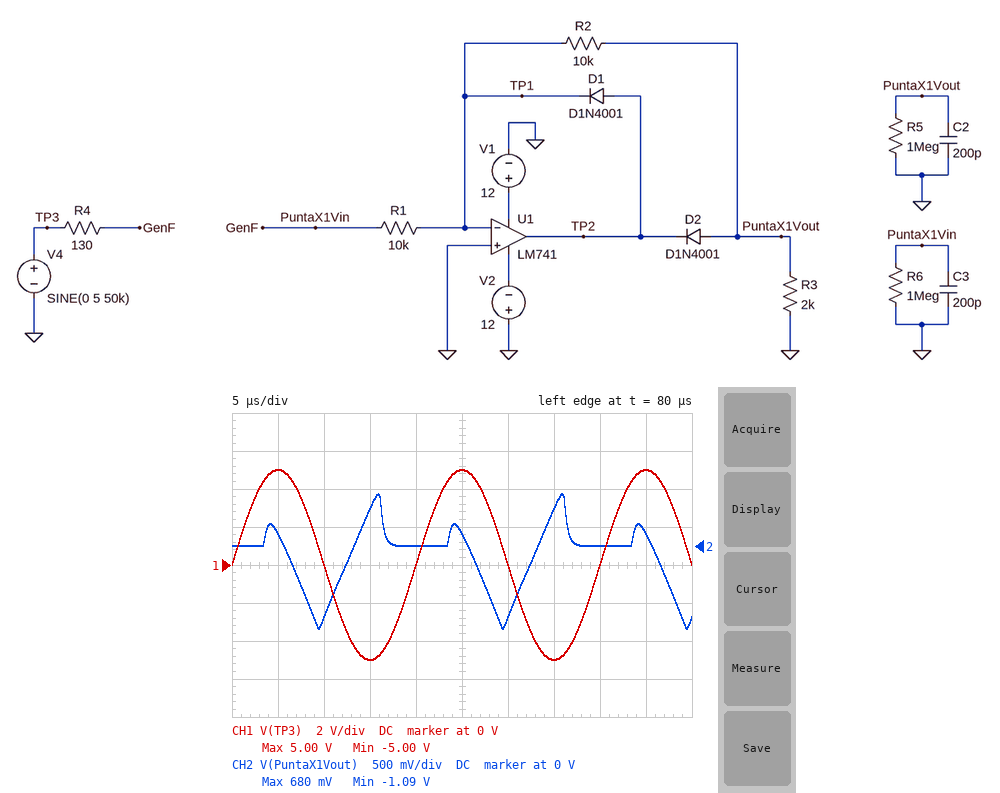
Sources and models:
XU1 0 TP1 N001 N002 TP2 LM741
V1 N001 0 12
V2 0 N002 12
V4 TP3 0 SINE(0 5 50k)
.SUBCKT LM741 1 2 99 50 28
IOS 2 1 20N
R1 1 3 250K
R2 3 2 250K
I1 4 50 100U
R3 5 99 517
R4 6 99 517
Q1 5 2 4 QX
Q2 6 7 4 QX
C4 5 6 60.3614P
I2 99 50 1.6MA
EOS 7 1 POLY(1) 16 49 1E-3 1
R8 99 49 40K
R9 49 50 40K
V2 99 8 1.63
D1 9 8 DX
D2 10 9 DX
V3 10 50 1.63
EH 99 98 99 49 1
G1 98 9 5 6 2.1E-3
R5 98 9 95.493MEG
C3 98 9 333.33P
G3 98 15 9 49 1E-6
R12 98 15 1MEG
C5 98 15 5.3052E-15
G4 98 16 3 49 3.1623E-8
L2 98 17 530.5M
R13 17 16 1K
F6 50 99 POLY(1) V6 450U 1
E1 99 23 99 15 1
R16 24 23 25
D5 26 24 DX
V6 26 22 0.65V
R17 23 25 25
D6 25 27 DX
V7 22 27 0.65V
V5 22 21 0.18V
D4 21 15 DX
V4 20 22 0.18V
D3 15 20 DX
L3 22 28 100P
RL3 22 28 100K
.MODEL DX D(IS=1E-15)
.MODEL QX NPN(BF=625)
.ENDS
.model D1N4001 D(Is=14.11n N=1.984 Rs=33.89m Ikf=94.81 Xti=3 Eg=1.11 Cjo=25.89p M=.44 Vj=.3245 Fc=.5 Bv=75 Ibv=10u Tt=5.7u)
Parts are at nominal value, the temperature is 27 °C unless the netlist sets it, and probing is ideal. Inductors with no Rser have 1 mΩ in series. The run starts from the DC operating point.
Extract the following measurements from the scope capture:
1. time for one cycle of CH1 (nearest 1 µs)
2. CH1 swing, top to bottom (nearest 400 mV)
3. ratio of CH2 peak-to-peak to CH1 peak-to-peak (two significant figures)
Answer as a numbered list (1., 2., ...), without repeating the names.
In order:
1. 20 µs
2. 10.0 V
3. 0.18
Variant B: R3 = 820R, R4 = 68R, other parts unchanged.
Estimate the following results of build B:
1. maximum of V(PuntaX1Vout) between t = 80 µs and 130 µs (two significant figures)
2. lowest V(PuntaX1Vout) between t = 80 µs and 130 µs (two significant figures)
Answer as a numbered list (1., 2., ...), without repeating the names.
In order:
1. 720 mV
2. -1.0 V
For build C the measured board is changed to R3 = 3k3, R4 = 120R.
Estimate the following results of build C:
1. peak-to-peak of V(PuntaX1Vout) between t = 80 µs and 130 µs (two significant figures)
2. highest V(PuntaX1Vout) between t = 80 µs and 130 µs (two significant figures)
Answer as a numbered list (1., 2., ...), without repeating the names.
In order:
1. 1.7 V
2. 630 mV
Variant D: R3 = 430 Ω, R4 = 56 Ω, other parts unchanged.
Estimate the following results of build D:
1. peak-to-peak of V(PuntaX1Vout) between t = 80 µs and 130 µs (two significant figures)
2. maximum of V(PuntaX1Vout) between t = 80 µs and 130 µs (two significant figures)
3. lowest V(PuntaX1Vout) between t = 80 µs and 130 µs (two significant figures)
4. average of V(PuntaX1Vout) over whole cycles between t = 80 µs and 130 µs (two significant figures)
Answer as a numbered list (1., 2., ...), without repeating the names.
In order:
1. 1.7 V
2. 710 mV
3. -990 mV
4. -110 mV
